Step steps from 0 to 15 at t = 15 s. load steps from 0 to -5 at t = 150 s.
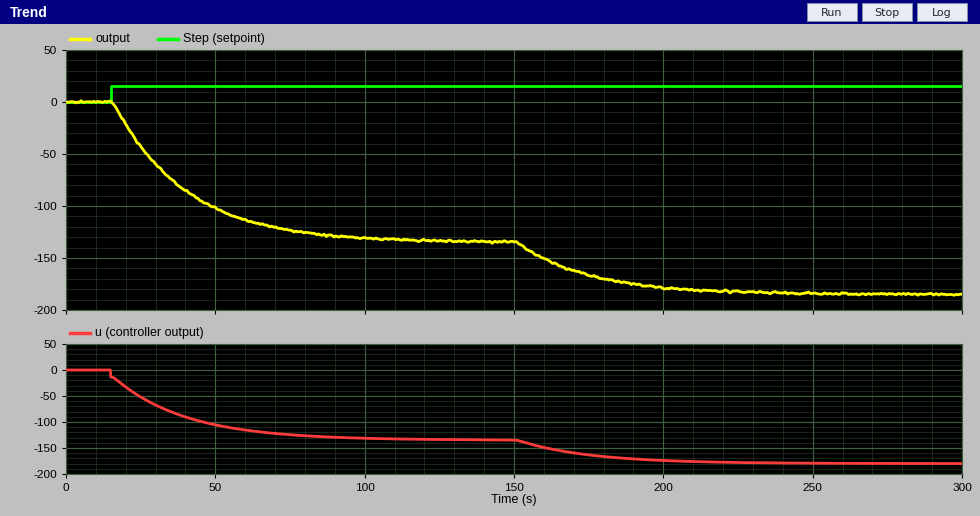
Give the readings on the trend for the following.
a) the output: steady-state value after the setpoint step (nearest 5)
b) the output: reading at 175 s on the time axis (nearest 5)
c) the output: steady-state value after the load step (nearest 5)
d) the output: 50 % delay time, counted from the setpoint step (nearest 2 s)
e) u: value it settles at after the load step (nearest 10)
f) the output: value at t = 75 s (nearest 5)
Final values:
-135
-165
-185
18 s
-180
-125
